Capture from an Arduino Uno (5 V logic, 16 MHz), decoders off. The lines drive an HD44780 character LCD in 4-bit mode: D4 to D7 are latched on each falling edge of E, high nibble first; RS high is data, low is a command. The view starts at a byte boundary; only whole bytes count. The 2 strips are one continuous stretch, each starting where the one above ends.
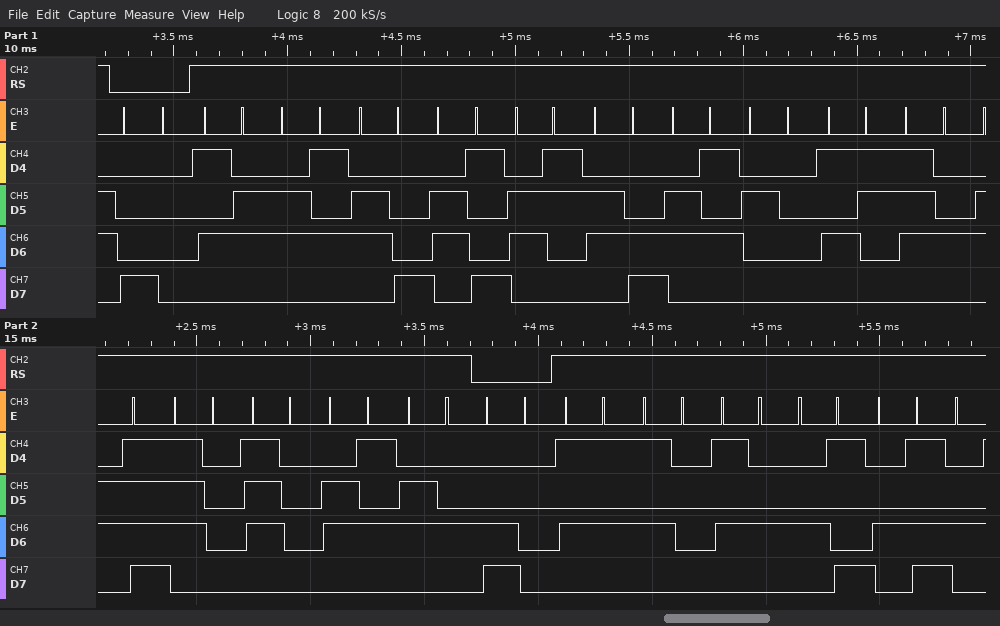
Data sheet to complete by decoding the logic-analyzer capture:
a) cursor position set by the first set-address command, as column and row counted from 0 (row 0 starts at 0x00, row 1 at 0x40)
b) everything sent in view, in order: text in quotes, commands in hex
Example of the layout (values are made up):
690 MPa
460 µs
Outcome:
column 0, row 0
0x80 "Vehicle Stopped" 0xC0 "UPTIM"
